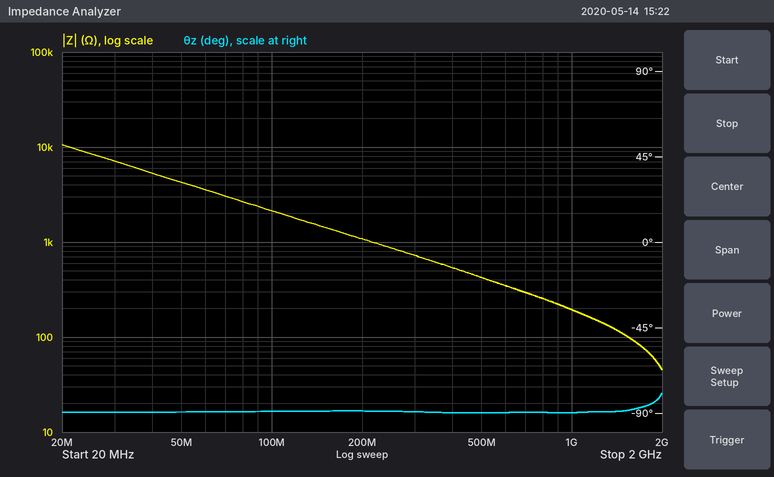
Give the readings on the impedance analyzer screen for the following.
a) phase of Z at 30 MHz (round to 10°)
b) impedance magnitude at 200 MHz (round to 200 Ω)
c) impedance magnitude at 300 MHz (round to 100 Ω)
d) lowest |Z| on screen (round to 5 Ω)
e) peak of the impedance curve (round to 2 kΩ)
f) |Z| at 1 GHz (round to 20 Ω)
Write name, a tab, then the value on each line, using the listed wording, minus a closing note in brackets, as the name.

phase of Z at 30 MHz	-90°
impedance magnitude at 200 MHz	1.0 kΩ
impedance magnitude at 300 MHz	700 Ω
lowest |Z| on screen	45 Ω
peak of the impedance curve	10 kΩ
|Z| at 1 GHz	200 Ω
